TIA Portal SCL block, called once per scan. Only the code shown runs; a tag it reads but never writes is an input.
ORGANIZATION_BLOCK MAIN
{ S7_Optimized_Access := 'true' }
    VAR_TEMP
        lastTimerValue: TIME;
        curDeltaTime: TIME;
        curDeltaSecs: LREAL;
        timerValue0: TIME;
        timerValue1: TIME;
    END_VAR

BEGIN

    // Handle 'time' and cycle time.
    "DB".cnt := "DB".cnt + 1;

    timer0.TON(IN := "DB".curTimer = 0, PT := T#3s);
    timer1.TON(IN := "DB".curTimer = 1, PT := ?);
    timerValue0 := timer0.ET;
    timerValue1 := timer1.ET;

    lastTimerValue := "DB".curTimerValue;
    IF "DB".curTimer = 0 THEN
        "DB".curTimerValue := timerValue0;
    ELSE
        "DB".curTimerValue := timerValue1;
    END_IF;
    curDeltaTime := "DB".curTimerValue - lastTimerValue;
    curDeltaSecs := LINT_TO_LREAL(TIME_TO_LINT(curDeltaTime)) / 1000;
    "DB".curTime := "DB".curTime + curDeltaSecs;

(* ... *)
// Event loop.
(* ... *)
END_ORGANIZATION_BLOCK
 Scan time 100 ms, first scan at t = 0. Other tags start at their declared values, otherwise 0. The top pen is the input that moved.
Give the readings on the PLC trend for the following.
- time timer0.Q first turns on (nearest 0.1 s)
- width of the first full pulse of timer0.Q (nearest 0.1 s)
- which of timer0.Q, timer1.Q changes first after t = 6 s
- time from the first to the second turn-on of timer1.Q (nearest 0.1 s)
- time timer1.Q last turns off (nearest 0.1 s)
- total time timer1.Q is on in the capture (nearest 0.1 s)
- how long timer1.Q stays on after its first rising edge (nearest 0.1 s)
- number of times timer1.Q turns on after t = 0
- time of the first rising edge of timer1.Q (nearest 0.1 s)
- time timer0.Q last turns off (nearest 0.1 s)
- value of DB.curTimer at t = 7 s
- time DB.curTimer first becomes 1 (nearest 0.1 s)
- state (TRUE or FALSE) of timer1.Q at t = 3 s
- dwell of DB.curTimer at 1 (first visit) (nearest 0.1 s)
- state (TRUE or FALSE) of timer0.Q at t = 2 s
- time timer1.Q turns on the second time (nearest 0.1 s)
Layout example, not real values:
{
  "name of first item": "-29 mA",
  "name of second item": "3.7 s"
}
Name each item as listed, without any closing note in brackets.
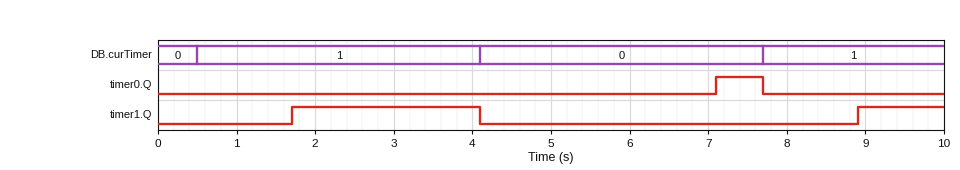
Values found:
{
  "time timer0.Q first turns on": "7.1 s",
  "width of the first full pulse of timer0.Q": "0.6 s",
  "which of timer0.Q, timer1.Q changes first after t = 6 s": "timer0.Q",
  "time from the first to the second turn-on of timer1.Q": "7.2 s",
  "time timer1.Q last turns off": "4.1 s",
  "total time timer1.Q is on in the capture": "3.5 s",
  "how long timer1.Q stays on after its first rising edge": "2.4 s",
  "number of times timer1.Q turns on after t = 0": "2",
  "time of the first rising edge of timer1.Q": "1.7 s",
  "time timer0.Q last turns off": "7.7 s",
  "value of DB.curTimer at t = 7 s": "0",
  "time DB.curTimer first becomes 1": "0.5 s",
  "state (TRUE or FALSE) of timer1.Q at t = 3 s": "TRUE",
  "dwell of DB.curTimer at 1 (first visit)": "3.6 s",
  "state (TRUE or FALSE) of timer0.Q at t = 2 s": "FALSE",
  "time timer1.Q turns on the second time": "8.9 s"
}
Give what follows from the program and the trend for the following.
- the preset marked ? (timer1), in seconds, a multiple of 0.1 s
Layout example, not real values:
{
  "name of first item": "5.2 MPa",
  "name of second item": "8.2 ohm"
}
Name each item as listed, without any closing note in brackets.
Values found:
{
  "the preset marked ? (timer1), in seconds, a multiple of 0.1 s": "1.2 s"
}
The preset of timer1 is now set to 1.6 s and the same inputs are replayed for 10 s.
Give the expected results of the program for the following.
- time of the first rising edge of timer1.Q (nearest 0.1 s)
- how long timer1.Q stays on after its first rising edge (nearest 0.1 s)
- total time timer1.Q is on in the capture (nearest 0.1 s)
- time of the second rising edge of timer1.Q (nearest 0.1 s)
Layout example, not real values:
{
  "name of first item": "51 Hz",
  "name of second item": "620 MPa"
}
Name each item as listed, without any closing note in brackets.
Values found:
{
  "time of the first rising edge of timer1.Q": "2.1 s",
  "how long timer1.Q stays on after its first rising edge": "2.0 s",
  "total time timer1.Q is on in the capture": "2.7 s",
  "time of the second rising edge of timer1.Q": "9.3 s"
}
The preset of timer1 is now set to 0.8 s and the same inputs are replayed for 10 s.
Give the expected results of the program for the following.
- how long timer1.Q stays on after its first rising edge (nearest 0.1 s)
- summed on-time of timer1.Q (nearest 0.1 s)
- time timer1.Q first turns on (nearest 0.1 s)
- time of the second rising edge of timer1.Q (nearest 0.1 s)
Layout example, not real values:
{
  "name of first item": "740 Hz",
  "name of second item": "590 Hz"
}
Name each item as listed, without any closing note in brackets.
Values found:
{
  "how long timer1.Q stays on after its first rising edge": "2.8 s",
  "summed on-time of timer1.Q": "4.3 s",
  "time timer1.Q first turns on": "1.3 s",
  "time of the second rising edge of timer1.Q": "8.5 s"
}
